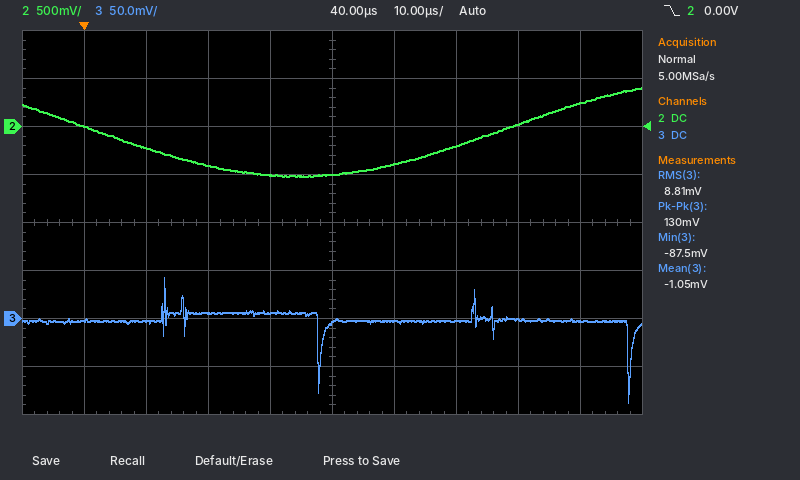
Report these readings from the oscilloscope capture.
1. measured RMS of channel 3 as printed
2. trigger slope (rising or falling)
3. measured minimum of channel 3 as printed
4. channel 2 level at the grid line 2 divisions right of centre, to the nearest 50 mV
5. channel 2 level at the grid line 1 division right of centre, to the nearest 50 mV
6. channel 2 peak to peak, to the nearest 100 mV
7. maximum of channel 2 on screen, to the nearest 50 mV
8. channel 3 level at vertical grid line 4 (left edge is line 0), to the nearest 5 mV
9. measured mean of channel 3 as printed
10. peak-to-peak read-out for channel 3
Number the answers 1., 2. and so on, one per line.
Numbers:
1. 8.81 mV
2. falling
3. -87.5 mV
4. -200 mV
5. -400 mV
6. 900 mV
7. 400 mV
8. 5 mV
9. -1.05 mV
10. 130 mV
